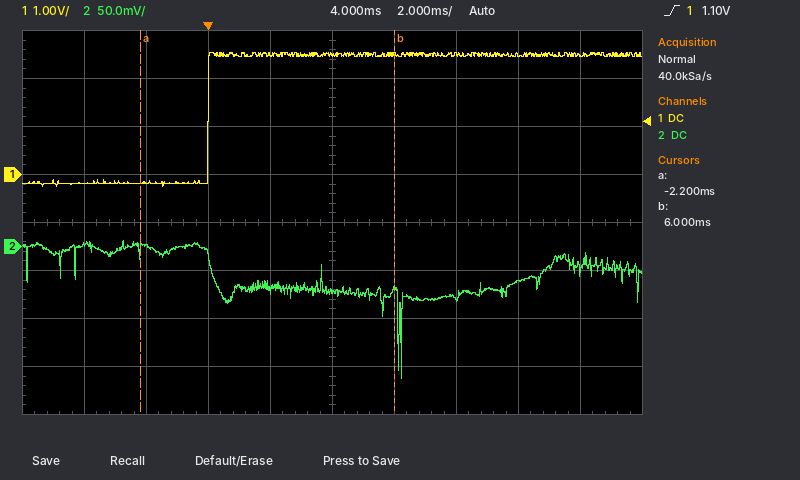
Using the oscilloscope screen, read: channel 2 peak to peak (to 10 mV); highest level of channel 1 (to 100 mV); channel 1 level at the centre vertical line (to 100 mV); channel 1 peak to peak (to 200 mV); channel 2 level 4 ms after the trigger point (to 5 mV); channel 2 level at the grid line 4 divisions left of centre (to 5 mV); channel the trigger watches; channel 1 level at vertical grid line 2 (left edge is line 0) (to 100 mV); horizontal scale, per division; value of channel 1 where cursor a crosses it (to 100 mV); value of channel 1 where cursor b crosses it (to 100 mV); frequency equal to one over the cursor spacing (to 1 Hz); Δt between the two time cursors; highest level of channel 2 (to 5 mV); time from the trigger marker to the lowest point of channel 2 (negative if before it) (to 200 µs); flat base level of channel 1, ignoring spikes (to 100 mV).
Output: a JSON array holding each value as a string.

["140 mV", "2.5 V", "2.5 V", "2.8 V", "-45 mV", "5 mV", "channel 1", "-200 mV", "2 ms", "-200 mV", "2.5 V", "122 Hz", "8.2 ms", "5 mV", "+6.2 ms", "-200 mV"]
